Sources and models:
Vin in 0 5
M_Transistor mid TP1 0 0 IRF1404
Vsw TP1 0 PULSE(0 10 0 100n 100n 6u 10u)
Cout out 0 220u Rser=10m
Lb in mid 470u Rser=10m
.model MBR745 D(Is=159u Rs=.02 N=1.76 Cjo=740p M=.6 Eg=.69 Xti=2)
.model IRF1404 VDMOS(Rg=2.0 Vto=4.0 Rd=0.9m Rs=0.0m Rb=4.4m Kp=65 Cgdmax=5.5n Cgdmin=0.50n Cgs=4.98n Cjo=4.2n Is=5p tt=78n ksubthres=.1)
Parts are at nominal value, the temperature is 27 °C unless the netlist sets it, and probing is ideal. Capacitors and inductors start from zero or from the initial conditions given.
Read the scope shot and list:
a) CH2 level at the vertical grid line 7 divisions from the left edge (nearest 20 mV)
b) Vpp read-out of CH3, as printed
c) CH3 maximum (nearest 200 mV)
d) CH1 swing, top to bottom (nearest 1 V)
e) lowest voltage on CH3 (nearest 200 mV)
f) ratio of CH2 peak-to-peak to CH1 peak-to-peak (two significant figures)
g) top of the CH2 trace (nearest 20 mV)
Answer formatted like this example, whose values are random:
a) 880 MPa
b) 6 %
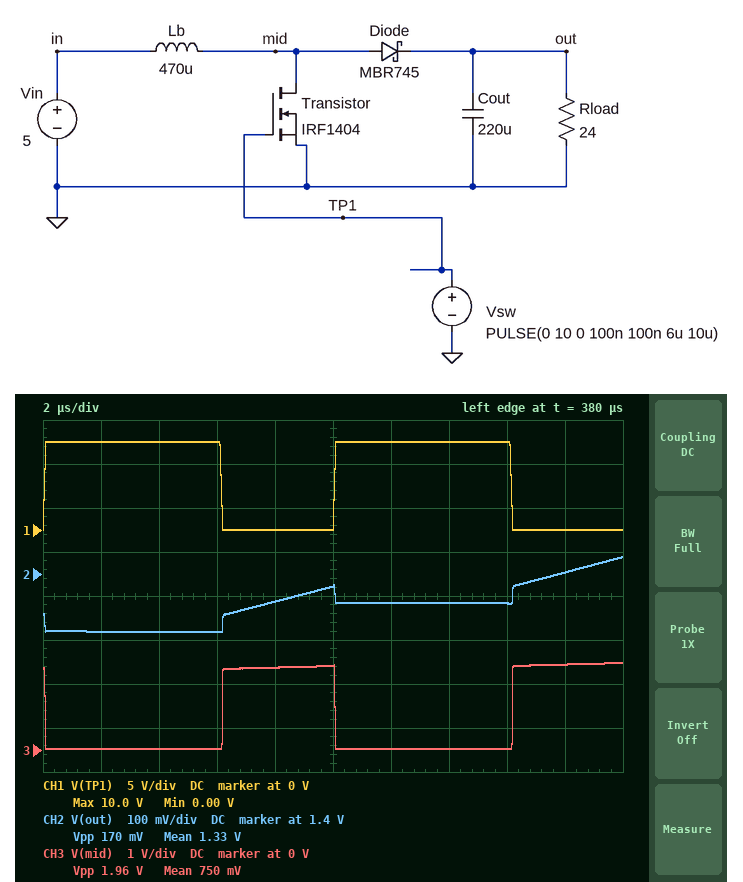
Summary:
a) 1.34 V
b) 1.96 V
c) 2.0 V
d) 10 V
e) 0 V
f) 0.017
g) 1.44 V
